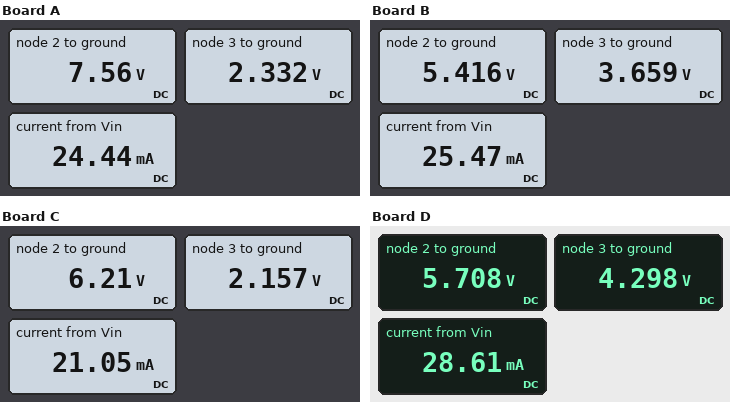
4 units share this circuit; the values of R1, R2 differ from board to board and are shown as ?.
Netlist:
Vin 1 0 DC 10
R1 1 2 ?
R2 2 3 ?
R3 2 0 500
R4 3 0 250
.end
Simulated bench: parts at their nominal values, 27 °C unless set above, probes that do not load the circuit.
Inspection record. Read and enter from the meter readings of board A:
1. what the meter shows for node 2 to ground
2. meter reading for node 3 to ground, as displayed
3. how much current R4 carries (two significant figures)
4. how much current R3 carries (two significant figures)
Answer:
7.56 V
2.332 V
9.3 mA
15 mA
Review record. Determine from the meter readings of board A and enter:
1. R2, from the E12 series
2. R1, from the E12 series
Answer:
560 Ω
100 Ω
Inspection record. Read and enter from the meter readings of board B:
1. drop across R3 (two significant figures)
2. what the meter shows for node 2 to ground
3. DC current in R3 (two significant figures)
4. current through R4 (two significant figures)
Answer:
5.4 V
5.416 V
11 mA
15 mA
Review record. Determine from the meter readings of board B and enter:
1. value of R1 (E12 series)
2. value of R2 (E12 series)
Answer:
180 Ω
120 Ω
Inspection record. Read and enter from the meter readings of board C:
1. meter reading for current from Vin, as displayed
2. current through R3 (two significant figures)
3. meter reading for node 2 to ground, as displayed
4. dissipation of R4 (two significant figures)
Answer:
21.05 mA
12 mA
6.21 V
19 mW
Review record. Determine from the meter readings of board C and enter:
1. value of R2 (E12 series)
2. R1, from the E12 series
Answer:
470 Ω
180 Ω
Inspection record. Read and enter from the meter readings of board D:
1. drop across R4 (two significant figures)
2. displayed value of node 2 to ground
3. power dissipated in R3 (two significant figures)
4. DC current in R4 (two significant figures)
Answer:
4.3 V
5.708 V
65 mW
17 mA
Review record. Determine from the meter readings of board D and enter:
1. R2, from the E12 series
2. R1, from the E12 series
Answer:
82 Ω
150 Ω
